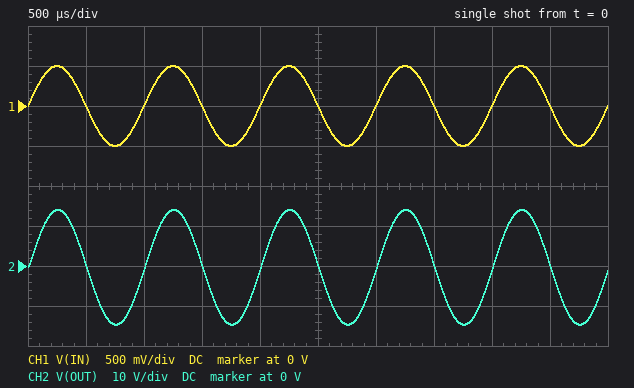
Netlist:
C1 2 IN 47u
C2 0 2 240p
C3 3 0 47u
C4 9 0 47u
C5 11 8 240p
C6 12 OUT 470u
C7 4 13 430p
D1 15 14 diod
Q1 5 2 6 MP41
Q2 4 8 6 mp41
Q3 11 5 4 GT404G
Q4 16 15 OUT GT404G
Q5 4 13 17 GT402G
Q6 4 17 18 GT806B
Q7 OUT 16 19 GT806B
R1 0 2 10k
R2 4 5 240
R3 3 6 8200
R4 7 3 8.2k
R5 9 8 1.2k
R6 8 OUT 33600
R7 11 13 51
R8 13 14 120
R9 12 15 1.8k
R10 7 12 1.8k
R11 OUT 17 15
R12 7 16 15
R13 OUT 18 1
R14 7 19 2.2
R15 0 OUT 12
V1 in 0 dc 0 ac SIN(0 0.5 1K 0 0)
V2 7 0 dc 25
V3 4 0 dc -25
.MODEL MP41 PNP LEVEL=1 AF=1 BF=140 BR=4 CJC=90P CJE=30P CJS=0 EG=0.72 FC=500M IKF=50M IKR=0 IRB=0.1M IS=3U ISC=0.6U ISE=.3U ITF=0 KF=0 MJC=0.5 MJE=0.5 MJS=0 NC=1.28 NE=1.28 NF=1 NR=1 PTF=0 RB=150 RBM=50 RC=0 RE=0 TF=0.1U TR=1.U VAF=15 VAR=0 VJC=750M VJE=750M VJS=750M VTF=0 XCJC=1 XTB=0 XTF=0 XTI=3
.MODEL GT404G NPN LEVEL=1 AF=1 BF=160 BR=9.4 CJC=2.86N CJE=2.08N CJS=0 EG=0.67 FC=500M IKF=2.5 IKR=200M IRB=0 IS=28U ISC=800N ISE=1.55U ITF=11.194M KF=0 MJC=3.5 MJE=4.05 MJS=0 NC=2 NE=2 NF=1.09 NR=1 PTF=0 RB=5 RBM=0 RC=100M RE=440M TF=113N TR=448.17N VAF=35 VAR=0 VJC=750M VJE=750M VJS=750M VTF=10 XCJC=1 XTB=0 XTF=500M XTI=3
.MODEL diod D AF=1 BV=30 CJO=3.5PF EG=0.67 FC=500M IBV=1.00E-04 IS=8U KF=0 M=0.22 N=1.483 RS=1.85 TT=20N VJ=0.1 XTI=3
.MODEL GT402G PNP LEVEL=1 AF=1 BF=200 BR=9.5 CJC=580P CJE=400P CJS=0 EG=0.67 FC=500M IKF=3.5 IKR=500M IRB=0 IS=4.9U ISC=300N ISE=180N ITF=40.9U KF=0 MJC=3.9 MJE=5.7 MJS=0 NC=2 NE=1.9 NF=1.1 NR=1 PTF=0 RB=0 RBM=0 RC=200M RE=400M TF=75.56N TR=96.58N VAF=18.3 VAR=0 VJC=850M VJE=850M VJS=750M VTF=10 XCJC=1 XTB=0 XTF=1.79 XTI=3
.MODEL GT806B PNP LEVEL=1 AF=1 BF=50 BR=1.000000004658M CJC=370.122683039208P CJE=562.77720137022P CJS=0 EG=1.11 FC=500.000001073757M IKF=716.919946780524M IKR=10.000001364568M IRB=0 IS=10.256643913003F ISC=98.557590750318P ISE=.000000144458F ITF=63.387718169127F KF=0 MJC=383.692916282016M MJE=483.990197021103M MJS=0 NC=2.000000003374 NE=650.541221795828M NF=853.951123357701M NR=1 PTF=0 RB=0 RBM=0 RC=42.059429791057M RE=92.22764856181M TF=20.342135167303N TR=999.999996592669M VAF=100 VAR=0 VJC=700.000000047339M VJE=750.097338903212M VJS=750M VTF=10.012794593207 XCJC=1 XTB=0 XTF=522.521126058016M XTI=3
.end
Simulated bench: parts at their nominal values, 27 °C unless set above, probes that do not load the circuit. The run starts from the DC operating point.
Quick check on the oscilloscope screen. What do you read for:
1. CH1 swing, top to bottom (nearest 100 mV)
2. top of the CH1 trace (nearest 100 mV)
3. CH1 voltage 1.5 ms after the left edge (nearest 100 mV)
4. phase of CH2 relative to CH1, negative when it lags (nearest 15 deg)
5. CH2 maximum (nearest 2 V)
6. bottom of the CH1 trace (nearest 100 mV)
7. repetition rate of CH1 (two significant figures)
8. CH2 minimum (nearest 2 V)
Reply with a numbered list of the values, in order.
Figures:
1. 1.0 V
2. 500 mV
3. 0 V
4. 0 deg
5. 14 V
6. -500 mV
7. 1.0 kHz
8. -14 V
